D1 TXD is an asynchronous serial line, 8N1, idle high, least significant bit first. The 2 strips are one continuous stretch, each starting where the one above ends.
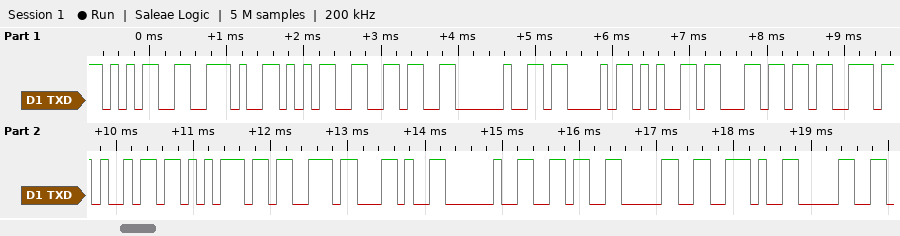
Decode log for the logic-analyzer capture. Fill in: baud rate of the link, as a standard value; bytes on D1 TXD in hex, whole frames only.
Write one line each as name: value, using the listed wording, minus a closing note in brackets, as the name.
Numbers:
baud rate of the link, as a standard value: 9600 baud
bytes on D1 TXD in hex, whole frames only: 35 2E 35 36 20 43 65 6C 73 69 75 73 2C 20 36 30 2E 30
